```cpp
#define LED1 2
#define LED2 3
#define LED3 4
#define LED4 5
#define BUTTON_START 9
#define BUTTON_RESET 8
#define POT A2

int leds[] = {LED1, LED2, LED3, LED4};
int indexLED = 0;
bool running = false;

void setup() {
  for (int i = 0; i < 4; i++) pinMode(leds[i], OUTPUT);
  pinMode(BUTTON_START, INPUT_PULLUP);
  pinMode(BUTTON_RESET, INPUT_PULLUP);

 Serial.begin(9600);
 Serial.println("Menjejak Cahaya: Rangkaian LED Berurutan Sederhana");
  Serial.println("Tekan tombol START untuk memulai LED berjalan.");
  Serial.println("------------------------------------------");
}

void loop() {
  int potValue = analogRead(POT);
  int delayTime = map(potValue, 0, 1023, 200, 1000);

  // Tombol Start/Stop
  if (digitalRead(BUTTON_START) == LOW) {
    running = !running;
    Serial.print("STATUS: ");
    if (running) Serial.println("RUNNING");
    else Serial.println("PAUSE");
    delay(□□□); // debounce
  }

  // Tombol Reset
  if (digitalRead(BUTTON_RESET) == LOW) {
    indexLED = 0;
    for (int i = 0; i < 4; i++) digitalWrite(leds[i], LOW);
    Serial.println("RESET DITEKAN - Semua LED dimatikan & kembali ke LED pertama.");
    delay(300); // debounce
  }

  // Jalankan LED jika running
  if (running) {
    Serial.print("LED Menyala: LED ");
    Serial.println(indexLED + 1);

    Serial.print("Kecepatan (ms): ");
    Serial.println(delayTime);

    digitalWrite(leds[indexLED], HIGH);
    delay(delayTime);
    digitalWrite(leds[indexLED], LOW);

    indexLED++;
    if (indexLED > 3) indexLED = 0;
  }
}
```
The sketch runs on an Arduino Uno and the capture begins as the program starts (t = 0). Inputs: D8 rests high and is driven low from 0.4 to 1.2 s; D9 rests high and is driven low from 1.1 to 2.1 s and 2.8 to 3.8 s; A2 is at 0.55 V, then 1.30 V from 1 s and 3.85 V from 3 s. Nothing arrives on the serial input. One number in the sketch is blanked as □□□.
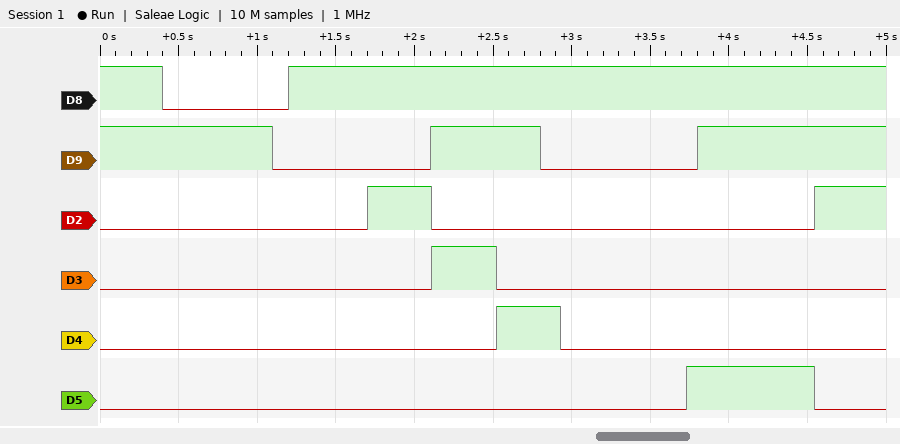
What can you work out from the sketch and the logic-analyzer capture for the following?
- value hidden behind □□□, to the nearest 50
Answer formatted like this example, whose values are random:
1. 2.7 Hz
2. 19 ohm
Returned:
1. 400
